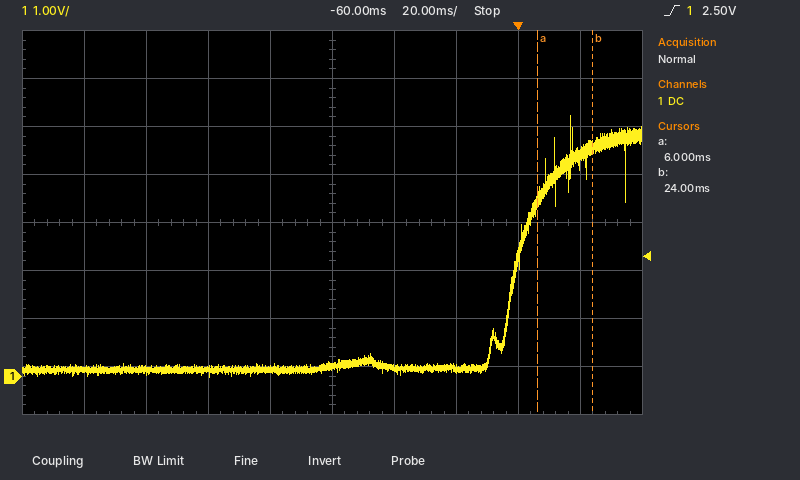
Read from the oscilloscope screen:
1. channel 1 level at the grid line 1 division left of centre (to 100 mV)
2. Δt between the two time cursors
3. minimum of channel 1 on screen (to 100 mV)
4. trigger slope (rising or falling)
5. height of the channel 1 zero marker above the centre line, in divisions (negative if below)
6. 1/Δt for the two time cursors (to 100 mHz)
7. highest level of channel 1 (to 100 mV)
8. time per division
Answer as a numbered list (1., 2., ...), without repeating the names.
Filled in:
1. 100 mV
2. 18 ms
3. 0.0 V
4. rising
5. -3.2 div
6. 55.6 Hz
7. 5.4 V
8. 20 ms
